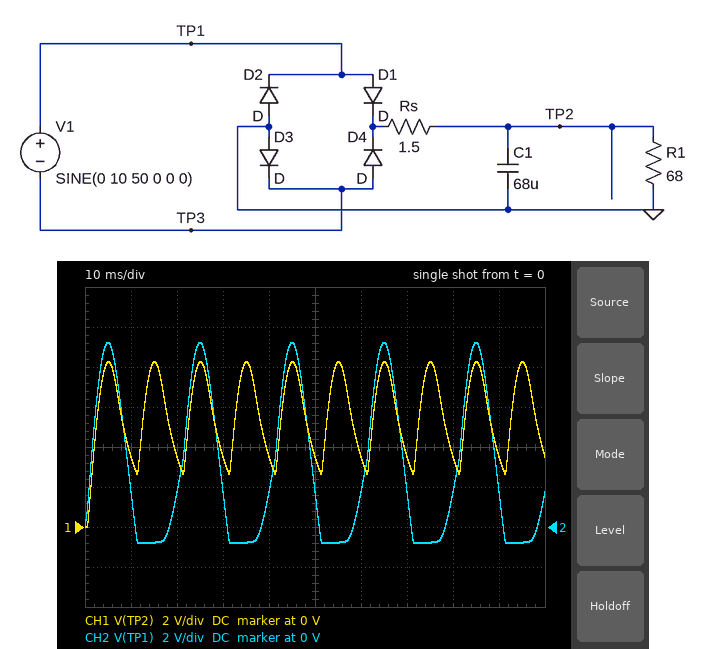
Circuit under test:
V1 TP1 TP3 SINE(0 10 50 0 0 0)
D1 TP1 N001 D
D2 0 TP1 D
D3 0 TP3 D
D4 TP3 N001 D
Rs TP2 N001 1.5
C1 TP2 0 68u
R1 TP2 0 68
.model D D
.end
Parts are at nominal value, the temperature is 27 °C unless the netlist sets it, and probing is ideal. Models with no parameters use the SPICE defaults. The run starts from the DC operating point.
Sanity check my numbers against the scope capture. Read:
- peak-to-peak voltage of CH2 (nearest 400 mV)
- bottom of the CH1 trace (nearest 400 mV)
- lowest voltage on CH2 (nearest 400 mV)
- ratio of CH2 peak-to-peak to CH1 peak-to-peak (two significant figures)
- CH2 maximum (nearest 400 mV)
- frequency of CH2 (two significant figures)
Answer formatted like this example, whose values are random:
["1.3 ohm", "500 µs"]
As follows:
["10.0 V", "0 V", "-800 mV", "1.2", "9.2 V", "50 Hz"]
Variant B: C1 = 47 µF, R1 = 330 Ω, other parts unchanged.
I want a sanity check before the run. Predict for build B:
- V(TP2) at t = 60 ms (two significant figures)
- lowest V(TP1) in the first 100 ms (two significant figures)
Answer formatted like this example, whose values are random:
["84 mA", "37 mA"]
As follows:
["6.3 V", "-780 mV"]
